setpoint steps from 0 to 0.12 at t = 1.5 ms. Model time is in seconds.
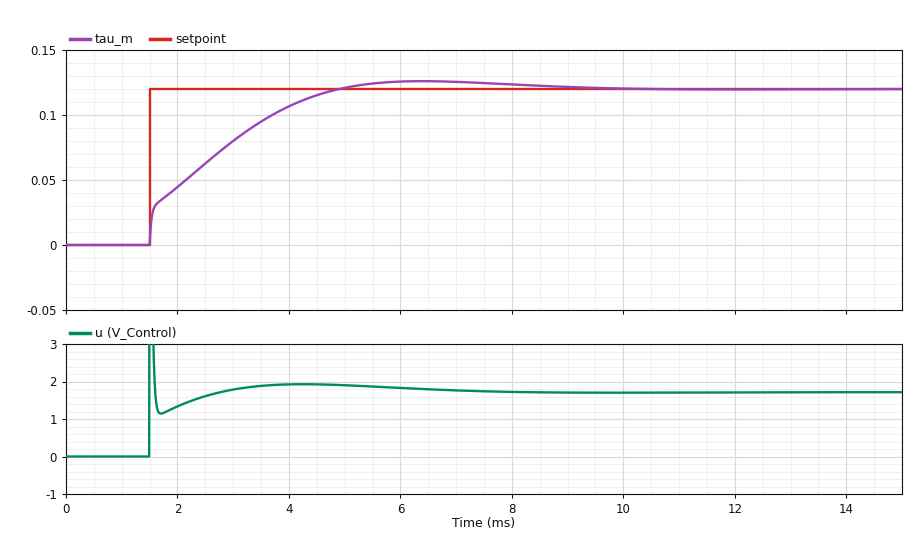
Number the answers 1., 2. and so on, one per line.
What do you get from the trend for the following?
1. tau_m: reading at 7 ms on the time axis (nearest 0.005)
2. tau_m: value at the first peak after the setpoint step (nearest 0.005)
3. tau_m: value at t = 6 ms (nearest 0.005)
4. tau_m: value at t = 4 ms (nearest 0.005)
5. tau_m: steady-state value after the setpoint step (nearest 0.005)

1. 0.125
2. 0.125
3. 0.125
4. 0.105
5. 0.120
